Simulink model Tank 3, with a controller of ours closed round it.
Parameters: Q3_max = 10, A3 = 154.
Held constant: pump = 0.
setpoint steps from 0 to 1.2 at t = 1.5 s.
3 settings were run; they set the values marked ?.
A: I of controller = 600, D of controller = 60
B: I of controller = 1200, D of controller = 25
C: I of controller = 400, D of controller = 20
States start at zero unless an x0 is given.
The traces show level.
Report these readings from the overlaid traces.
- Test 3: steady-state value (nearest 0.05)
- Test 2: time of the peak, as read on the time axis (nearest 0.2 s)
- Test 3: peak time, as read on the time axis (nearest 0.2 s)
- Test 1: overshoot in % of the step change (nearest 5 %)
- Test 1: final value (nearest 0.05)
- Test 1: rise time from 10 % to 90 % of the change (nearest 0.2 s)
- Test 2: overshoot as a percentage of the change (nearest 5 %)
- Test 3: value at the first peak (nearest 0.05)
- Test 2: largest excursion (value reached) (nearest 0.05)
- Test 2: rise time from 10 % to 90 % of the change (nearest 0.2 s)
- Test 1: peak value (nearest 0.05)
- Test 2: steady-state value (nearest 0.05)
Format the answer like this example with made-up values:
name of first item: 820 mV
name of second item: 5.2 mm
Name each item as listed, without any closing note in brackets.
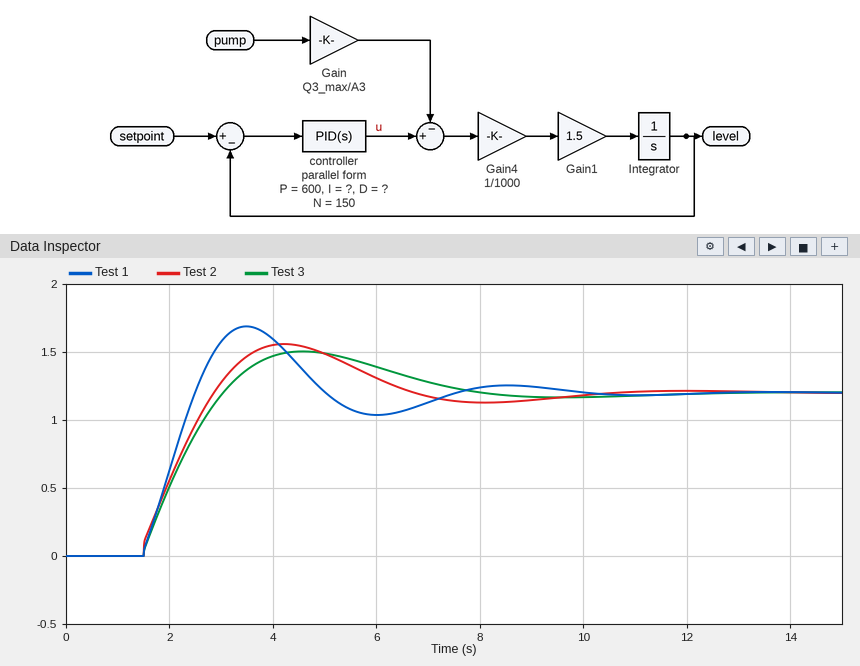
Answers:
Test 3: steady-state value: 1.20
Test 2: time of the peak, as read on the time axis: 4.2 s
Test 3: peak time, as read on the time axis: 4.6 s
Test 1: overshoot in % of the step change: 40 %
Test 1: final value: 1.20
Test 1: rise time from 10 % to 90 % of the change: 0.8 s
Test 2: overshoot as a percentage of the change: 30 %
Test 3: value at the first peak: 1.50
Test 2: largest excursion (value reached): 1.55
Test 2: rise time from 10 % to 90 % of the change: 1.2 s
Test 1: peak value: 1.70
Test 2: steady-state value: 1.20
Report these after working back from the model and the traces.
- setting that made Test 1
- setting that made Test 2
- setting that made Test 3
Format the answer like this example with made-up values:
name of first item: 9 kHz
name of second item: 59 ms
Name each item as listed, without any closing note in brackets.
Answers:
setting that made Test 1: B
setting that made Test 2: A
setting that made Test 3: C
